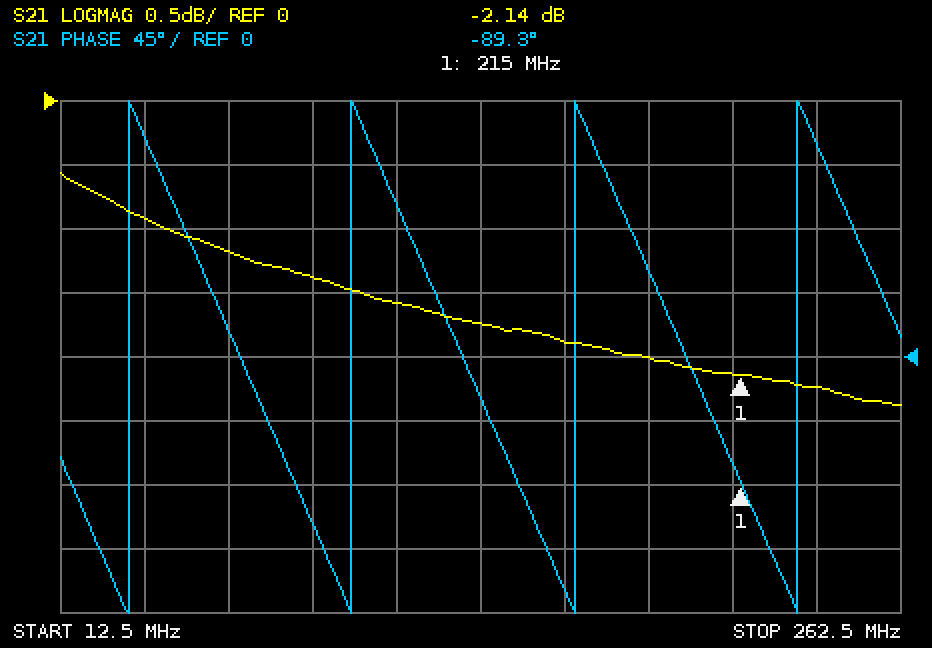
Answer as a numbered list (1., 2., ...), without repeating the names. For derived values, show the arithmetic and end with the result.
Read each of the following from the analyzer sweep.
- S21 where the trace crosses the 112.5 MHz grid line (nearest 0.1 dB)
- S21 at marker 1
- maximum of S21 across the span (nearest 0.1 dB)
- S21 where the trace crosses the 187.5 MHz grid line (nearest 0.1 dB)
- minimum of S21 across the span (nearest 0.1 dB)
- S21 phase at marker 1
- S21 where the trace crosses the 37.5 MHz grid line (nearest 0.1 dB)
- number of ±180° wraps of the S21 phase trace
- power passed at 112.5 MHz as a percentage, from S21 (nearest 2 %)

1. -1.6 dB
2. -2.14 dB
3. -0.6 dB
4. -2.0 dB
5. -2.4 dB
6. -89.3°
7. -0.9 dB
8. 4
9. 10^(-1.6/10) ≈ 69.2 %, so 70 % to the nearest 2 %
